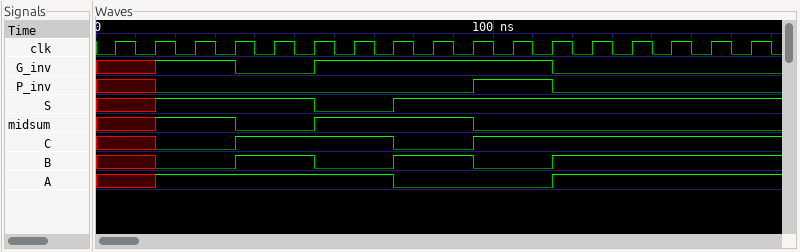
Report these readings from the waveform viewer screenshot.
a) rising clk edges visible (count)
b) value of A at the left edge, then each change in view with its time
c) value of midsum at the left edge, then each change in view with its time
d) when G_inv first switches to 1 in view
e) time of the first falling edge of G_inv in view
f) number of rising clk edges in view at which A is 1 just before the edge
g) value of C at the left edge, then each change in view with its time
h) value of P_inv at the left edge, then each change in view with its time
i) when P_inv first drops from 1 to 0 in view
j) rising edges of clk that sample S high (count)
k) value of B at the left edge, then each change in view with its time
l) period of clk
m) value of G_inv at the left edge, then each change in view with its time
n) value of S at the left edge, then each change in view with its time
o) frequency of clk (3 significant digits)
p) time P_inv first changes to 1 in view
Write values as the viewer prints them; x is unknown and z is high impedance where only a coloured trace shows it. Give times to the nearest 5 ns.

17
x, 1 at 15 ns, 0 at 75 ns, 1 at 115 ns
x, 1 at 15 ns, 0 at 35 ns, 1 at 55 ns, 0 at 95 ns
15 ns
35 ns
11
x, 0 at 15 ns, 1 at 35 ns, 0 at 75 ns, 1 at 95 ns
x, 0 at 15 ns, 1 at 95 ns, 0 at 115 ns
115 ns
13
x, 0 at 15 ns, 1 at 35 ns, 0 at 55 ns, 1 at 75 ns, 0 at 95 ns, 1 at 115 ns
10 ns
x, 1 at 15 ns, 0 at 35 ns, 1 at 55 ns, 0 at 115 ns
x, 1 at 15 ns, 0 at 55 ns, 1 at 75 ns
100 MHz
95 ns
